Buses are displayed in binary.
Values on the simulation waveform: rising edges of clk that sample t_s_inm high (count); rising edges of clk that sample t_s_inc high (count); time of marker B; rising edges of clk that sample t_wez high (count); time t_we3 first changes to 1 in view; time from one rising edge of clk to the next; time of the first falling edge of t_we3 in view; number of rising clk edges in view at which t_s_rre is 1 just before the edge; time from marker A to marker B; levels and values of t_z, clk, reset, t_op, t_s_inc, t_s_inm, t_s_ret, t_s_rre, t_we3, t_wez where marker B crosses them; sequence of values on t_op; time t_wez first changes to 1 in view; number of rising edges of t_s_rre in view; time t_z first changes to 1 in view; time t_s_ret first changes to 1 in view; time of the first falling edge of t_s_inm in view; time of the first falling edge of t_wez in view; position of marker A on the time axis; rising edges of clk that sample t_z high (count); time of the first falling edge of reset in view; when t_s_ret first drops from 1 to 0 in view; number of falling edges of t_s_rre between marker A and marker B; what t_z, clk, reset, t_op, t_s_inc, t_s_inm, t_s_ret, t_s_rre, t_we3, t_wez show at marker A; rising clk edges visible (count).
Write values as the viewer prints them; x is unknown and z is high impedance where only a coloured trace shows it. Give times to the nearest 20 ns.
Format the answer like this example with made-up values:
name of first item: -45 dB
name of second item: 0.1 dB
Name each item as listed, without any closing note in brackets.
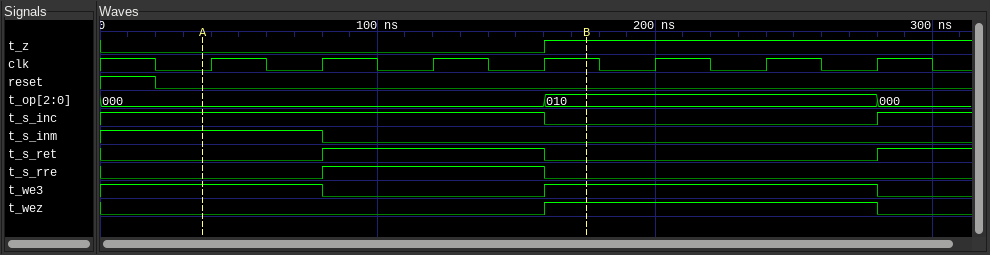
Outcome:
rising edges of clk that sample t_s_inm high: 2
rising edges of clk that sample t_s_inc high: 4
time of marker B: 180 ns
rising edges of clk that sample t_wez high: 3
time t_we3 first changes to 1 in view: 160 ns
time from one rising edge of clk to the next: 40 ns
time of the first falling edge of t_we3 in view: 80 ns
number of rising clk edges in view at which t_s_rre is 1 just before the edge: 2
time from marker A to marker B: 140 ns
levels and values of t_z, clk, reset, t_op, t_s_inc, t_s_inm, t_s_ret, t_s_rre, t_we3, t_wez where marker B crosses them: t_z=1, clk=1, reset=0, t_op=010, t_s_inc=0, t_s_inm=0, t_s_ret=0, t_s_rre=0, t_we3=1, t_wez=1
sequence of values on t_op: 000, 010, 000
time t_wez first changes to 1 in view: 160 ns
number of rising edges of t_s_rre in view: 1
time t_z first changes to 1 in view: 160 ns
time t_s_ret first changes to 1 in view: 80 ns
time of the first falling edge of t_s_inm in view: 80 ns
time of the first falling edge of t_wez in view: 280 ns
position of marker A on the time axis: 40 ns
rising edges of clk that sample t_z high: 3
time of the first falling edge of reset in view: 20 ns
when t_s_ret first drops from 1 to 0 in view: 160 ns
number of falling edges of t_s_rre between marker A and marker B: 1
what t_z, clk, reset, t_op, t_s_inc, t_s_inm, t_s_ret, t_s_rre, t_we3, t_wez show at marker A: t_z=0, clk=0, reset=0, t_op=000, t_s_inc=1, t_s_inm=1, t_s_ret=0, t_s_rre=0, t_we3=1, t_wez=0
rising clk edges visible: 7
